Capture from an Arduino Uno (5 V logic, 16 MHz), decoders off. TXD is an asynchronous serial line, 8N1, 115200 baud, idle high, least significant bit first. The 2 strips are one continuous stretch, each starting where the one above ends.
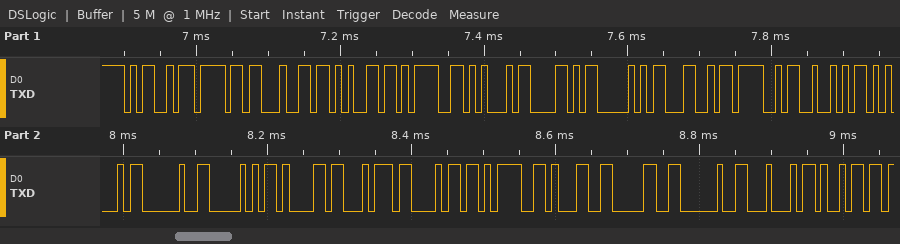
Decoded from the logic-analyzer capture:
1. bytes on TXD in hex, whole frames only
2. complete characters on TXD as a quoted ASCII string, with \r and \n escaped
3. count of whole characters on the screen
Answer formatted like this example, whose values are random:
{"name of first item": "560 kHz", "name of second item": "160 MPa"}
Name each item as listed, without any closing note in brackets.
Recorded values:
{"bytes on TXD in hex, whole frames only": "4D 6F 64 65 3D 45 58 50 4C 4F 52 45 20 50 61 74 68 3D 31 30 20 44 69", "complete characters on TXD as a quoted ASCII string, with \\r and \\n escaped": "\"Mode=EXPLORE Path=10 Di\"", "count of whole characters on the screen": "23"}
